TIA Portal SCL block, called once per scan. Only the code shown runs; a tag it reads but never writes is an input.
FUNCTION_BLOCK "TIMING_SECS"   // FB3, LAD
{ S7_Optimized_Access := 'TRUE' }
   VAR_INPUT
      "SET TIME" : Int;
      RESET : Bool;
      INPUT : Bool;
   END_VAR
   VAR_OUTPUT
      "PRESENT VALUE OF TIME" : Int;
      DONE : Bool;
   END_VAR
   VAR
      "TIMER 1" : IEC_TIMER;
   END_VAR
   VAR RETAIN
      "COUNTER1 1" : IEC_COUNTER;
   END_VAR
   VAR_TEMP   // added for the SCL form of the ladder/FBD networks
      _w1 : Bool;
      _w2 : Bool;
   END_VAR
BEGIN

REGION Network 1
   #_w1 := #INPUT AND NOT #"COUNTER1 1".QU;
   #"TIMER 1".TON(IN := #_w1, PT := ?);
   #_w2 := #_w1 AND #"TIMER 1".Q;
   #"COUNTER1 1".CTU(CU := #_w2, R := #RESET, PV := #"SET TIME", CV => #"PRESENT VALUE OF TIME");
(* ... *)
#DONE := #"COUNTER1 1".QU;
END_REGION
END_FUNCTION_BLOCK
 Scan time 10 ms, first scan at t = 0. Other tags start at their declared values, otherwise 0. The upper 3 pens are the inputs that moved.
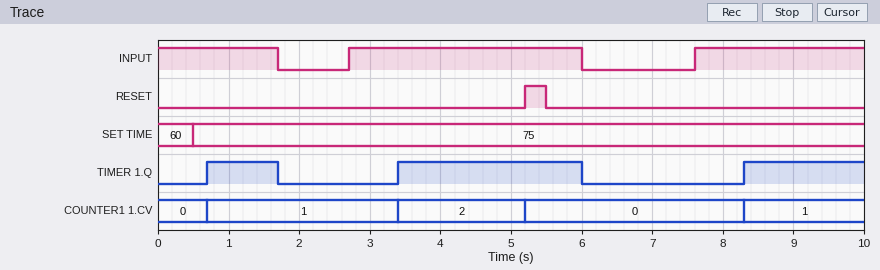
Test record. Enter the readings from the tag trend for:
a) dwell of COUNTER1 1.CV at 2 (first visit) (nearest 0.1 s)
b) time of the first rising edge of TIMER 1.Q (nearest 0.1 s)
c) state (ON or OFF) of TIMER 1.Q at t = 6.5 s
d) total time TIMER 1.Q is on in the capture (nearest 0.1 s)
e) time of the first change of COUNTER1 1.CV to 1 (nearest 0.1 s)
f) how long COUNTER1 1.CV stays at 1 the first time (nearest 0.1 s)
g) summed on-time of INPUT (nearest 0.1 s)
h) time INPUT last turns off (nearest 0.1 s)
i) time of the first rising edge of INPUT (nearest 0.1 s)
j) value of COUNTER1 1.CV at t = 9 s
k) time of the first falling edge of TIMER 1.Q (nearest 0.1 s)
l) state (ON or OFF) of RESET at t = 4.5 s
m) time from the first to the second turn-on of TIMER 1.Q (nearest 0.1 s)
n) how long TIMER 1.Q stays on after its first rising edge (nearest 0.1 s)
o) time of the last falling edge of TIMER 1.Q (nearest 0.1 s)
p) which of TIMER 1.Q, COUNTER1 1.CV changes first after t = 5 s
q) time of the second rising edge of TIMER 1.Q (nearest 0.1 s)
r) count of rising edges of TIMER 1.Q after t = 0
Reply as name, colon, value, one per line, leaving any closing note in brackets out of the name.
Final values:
dwell of COUNTER1 1.CV at 2 (first visit): 1.8 s
time of the first rising edge of TIMER 1.Q: 0.7 s
state (ON or OFF) of TIMER 1.Q at t = 6.5 s: OFF
total time TIMER 1.Q is on in the capture: 5.3 s
time of the first change of COUNTER1 1.CV to 1: 0.7 s
how long COUNTER1 1.CV stays at 1 the first time: 2.7 s
summed on-time of INPUT: 7.4 s
time INPUT last turns off: 6.0 s
time of the first rising edge of INPUT: 2.7 s
value of COUNTER1 1.CV at t = 9 s: 1
time of the first falling edge of TIMER 1.Q: 1.7 s
state (ON or OFF) of RESET at t = 4.5 s: OFF
time from the first to the second turn-on of TIMER 1.Q: 2.7 s
how long TIMER 1.Q stays on after its first rising edge: 1.0 s
time of the last falling edge of TIMER 1.Q: 6.0 s
which of TIMER 1.Q, COUNTER1 1.CV changes first after t = 5 s: COUNTER1 1.CV
time of the second rising edge of TIMER 1.Q: 3.4 s
count of rising edges of TIMER 1.Q after t = 0: 3
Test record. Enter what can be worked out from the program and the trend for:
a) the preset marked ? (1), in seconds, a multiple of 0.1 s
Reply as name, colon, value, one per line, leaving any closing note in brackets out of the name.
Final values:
the preset marked ? (1), in seconds, a multiple of 0.1 s: 0.7 s
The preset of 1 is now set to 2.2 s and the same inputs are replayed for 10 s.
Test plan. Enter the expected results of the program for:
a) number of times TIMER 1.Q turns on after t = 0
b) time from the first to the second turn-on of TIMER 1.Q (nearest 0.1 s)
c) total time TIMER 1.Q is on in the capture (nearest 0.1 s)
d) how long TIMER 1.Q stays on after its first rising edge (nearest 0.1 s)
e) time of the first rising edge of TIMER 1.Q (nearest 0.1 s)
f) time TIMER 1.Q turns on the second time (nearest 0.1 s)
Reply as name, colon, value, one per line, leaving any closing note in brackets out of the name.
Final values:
number of times TIMER 1.Q turns on after t = 0: 2
time from the first to the second turn-on of TIMER 1.Q: 4.9 s
total time TIMER 1.Q is on in the capture: 1.3 s
how long TIMER 1.Q stays on after its first rising edge: 1.1 s
time of the first rising edge of TIMER 1.Q: 4.9 s
time TIMER 1.Q turns on the second time: 9.8 s
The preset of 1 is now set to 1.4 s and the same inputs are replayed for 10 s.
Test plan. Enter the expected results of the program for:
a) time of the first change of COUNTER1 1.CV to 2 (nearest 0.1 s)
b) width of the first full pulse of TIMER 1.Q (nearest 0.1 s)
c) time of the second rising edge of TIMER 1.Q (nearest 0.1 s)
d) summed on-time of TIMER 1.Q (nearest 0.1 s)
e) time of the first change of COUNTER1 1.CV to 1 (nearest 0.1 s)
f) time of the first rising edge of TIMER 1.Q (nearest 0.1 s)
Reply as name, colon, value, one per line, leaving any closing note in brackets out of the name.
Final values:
time of the first change of COUNTER1 1.CV to 2: 4.1 s
width of the first full pulse of TIMER 1.Q: 0.3 s
time of the second rising edge of TIMER 1.Q: 4.1 s
summed on-time of TIMER 1.Q: 3.2 s
time of the first change of COUNTER1 1.CV to 1: 1.4 s
time of the first rising edge of TIMER 1.Q: 1.4 s
